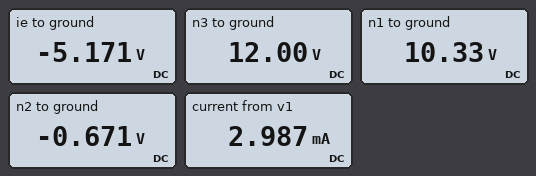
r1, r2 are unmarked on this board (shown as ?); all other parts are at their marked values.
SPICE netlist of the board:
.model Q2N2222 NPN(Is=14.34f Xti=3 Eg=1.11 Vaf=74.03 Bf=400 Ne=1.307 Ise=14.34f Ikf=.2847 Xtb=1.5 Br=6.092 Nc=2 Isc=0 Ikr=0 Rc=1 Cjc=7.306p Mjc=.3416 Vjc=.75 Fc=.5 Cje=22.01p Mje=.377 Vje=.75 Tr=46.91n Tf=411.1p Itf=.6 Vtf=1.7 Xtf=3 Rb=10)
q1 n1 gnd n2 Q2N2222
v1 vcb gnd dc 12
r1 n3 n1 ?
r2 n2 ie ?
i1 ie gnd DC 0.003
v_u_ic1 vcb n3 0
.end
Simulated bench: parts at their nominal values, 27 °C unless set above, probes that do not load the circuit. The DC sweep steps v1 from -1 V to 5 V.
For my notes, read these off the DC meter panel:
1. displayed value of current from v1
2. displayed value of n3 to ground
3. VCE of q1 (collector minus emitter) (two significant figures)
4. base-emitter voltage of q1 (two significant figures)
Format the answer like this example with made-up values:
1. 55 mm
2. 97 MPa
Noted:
1. 2.987 mA
2. 12.00 V
3. 11 V
4. 670 mV
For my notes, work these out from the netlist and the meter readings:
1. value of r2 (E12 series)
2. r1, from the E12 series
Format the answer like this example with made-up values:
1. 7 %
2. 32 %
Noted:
1. 1.5 kΩ
2. 560 Ω
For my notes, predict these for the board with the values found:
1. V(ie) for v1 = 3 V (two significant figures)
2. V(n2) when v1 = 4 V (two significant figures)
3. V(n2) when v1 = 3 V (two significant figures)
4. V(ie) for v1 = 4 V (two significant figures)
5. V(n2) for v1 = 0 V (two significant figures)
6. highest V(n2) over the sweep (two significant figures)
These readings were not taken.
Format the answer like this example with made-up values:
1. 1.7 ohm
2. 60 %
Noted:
1. -5.2 V
2. -670 mV
3. -670 mV
4. -5.2 V
5. -730 mV
6. -670 mV
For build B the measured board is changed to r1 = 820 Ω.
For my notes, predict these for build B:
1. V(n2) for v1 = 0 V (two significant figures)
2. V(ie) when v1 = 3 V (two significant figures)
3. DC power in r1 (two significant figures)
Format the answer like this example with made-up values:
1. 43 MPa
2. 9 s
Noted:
1. -740 mV
2. -5.2 V
3. 7.3 mW
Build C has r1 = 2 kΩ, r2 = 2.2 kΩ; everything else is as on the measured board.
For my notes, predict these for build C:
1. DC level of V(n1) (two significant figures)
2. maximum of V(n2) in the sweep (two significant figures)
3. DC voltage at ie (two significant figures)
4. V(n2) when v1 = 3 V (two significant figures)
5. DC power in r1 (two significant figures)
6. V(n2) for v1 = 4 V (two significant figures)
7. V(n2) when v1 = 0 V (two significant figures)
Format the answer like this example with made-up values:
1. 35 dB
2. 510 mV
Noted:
1. 6.0 V
2. -680 mV
3. -7.3 V
4. -720 mV
5. 18 mW
6. -700 mV
7. -750 mV
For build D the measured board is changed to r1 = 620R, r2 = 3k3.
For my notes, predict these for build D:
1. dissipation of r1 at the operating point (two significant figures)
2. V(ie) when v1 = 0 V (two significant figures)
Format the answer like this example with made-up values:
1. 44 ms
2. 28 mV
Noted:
1. 5.5 mW
2. -11 V
